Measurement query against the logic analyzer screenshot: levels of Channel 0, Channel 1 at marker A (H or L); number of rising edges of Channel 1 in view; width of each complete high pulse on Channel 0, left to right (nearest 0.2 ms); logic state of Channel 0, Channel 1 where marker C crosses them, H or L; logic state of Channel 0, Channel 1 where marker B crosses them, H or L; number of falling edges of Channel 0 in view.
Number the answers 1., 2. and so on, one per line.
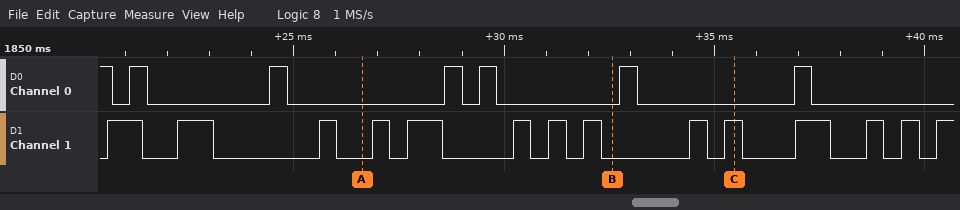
1. Channel 0=L, Channel 1=L
2. 14
3. 0.4 ms, 0.4 ms, 0.4 ms, 0.4 ms, 0.4 ms, 0.4 ms
4. Channel 0=L, Channel 1=H
5. Channel 0=L, Channel 1=L
6. 7
